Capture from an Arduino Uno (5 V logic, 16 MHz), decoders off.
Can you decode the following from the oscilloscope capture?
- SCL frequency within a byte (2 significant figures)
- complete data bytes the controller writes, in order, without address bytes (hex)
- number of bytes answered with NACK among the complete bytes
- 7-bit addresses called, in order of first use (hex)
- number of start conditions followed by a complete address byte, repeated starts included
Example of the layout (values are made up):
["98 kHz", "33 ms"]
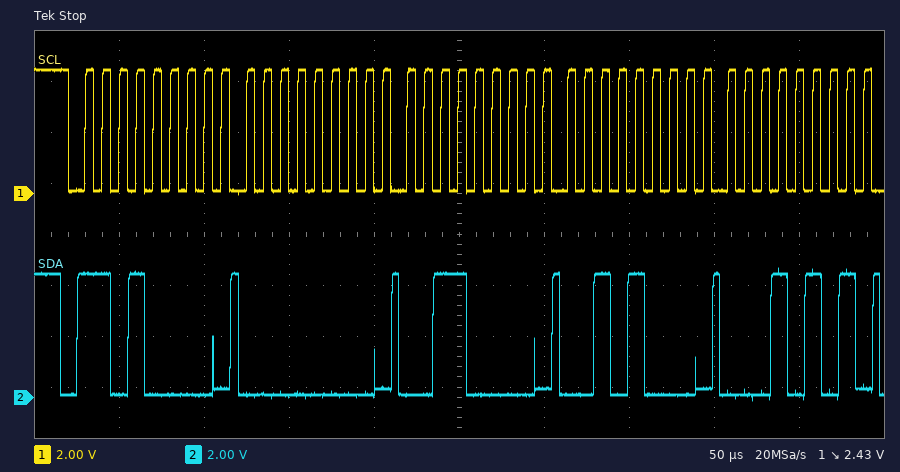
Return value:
["100 kHz", "00 30 28 15", "0", "0x68", "1"]
